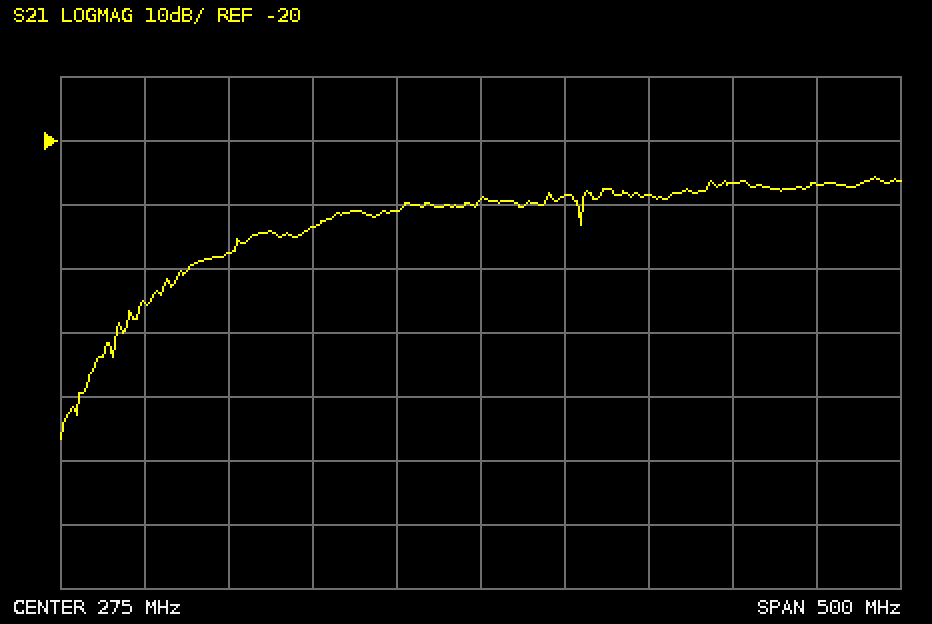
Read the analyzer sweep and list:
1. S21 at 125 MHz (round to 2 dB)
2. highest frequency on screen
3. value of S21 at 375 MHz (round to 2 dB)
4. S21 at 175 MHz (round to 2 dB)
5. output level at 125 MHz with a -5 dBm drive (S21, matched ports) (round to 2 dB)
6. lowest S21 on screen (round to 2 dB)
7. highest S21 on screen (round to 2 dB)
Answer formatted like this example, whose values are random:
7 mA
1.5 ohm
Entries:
-38 dB
525 MHz
-28 dB
-34 dB
-42 dBm
-66 dB
-26 dB
